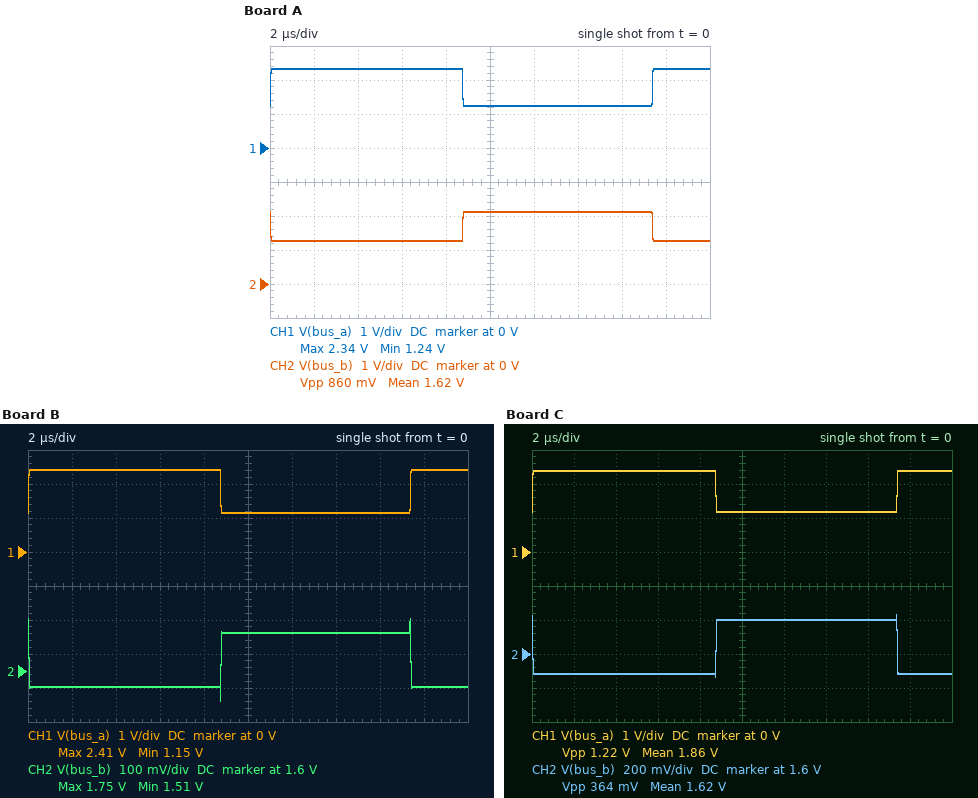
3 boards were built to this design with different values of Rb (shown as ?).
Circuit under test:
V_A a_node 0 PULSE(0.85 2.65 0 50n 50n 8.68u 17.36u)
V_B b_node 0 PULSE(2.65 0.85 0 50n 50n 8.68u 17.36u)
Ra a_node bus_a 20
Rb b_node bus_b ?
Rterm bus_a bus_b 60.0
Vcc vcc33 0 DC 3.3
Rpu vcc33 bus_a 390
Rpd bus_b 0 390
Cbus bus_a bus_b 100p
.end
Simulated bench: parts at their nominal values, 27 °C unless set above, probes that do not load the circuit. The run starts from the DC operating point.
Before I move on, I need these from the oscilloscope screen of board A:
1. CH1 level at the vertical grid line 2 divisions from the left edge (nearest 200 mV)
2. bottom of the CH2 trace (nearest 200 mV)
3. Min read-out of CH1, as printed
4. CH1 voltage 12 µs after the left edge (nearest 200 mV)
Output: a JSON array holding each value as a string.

["2.4 V", "1.2 V", "1.24 V", "1.2 V"]
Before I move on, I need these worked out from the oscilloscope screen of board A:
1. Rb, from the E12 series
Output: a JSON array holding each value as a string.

["27 Ω"]
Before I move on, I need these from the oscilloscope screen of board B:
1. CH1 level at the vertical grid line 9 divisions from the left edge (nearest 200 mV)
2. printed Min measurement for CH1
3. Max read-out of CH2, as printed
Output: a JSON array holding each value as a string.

["2.4 V", "1.15 V", "1.75 V"]
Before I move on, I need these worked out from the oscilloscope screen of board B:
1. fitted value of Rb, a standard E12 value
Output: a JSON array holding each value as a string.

["68 Ω"]
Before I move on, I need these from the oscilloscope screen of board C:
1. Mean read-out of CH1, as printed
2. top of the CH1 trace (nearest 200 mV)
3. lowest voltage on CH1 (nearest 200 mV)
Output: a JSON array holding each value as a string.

["1.86 V", "2.4 V", "1.2 V"]
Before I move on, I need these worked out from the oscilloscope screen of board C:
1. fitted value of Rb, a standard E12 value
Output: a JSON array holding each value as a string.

["56 Ω"]
